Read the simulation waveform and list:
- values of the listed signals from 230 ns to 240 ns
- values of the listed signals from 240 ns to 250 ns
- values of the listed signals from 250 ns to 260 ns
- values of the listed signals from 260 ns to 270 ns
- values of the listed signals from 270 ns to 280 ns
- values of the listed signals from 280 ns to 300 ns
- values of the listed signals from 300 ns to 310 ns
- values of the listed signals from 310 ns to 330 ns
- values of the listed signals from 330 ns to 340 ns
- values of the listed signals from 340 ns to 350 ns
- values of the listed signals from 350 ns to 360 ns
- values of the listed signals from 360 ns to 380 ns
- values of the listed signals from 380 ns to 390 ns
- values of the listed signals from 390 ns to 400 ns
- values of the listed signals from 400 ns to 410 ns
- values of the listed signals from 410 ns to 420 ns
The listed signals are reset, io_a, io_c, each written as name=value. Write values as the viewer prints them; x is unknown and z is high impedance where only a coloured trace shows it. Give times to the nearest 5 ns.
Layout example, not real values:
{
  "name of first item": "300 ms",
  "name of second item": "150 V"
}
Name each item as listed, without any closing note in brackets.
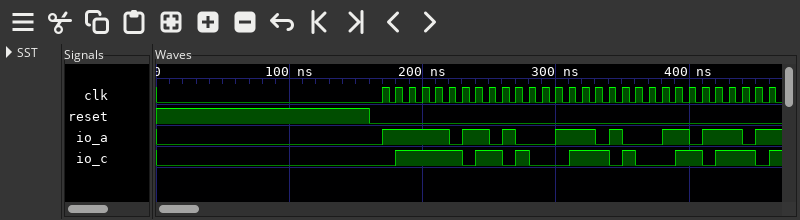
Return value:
{
  "values of the listed signals from 230 ns to 240 ns": "reset=0, io_a=1, io_c=0",
  "values of the listed signals from 240 ns to 250 ns": "reset=0, io_a=1, io_c=1",
  "values of the listed signals from 250 ns to 260 ns": "reset=0, io_a=0, io_c=1",
  "values of the listed signals from 260 ns to 270 ns": "reset=0, io_a=1, io_c=0",
  "values of the listed signals from 270 ns to 280 ns": "reset=0, io_a=0, io_c=1",
  "values of the listed signals from 280 ns to 300 ns": "reset=0, io_a=0, io_c=0",
  "values of the listed signals from 300 ns to 310 ns": "reset=0, io_a=1, io_c=0",
  "values of the listed signals from 310 ns to 330 ns": "reset=0, io_a=1, io_c=1",
  "values of the listed signals from 330 ns to 340 ns": "reset=0, io_a=0, io_c=1",
  "values of the listed signals from 340 ns to 350 ns": "reset=0, io_a=1, io_c=0",
  "values of the listed signals from 350 ns to 360 ns": "reset=0, io_a=0, io_c=1",
  "values of the listed signals from 360 ns to 380 ns": "reset=0, io_a=0, io_c=0",
  "values of the listed signals from 380 ns to 390 ns": "reset=0, io_a=1, io_c=0",
  "values of the listed signals from 390 ns to 400 ns": "reset=0, io_a=1, io_c=1",
  "values of the listed signals from 400 ns to 410 ns": "reset=0, io_a=0, io_c=1",
  "values of the listed signals from 410 ns to 420 ns": "reset=0, io_a=1, io_c=0"
}
